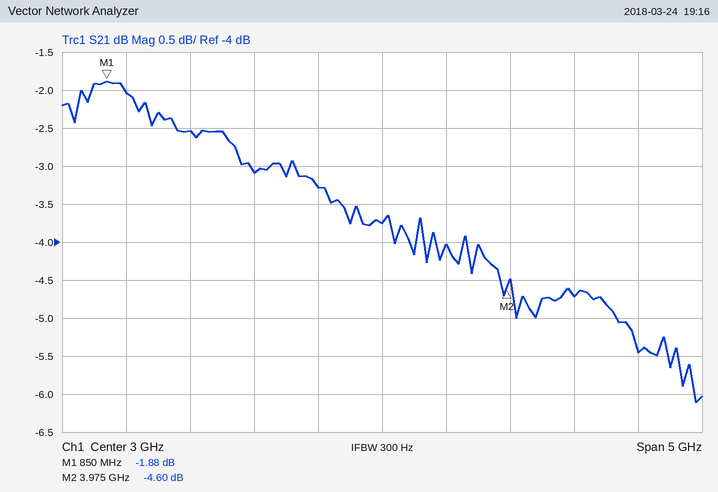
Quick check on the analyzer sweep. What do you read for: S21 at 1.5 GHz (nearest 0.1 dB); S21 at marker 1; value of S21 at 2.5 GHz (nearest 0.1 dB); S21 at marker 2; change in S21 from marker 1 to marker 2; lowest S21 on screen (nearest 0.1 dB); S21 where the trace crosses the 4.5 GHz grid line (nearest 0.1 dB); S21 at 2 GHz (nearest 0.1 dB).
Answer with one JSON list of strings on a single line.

["-2.5 dB", "-1.88 dB", "-3.3 dB", "-4.60 dB", "-2.72 dB", "-6.1 dB", "-4.7 dB", "-3.1 dB"]
